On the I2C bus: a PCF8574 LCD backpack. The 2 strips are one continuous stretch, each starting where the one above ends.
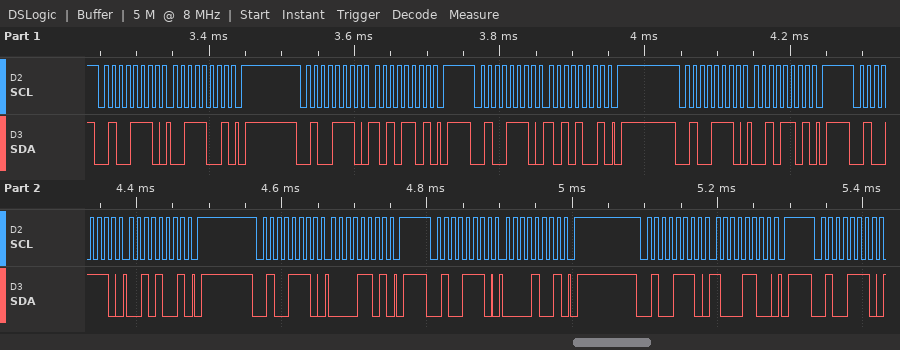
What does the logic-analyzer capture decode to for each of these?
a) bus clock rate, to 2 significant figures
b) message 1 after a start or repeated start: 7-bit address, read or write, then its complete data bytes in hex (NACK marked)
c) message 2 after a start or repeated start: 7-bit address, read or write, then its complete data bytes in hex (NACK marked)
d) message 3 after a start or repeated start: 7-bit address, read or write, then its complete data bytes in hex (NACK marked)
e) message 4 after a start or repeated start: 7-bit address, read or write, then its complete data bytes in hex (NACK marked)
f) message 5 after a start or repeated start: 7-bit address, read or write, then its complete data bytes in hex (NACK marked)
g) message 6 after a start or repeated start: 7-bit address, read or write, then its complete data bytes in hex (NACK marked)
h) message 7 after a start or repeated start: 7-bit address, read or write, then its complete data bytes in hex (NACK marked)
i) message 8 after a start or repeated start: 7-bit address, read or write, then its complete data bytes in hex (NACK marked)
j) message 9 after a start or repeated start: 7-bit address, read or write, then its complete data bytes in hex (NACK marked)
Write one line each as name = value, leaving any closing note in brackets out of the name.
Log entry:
bus clock rate, to 2 significant figures = 100 kHz
message 1 after a start or repeated start: 7-bit address, read or write, then its complete data bytes in hex = 0x27 write: 39
message 2 after a start or repeated start: 7-bit address, read or write, then its complete data bytes in hex = 0x27 write: AD
message 3 after a start or repeated start: 7-bit address, read or write, then its complete data bytes in hex = 0x27 write: A9
message 4 after a start or repeated start: 7-bit address, read or write, then its complete data bytes in hex = 0x27 write: 2D
message 5 after a start or repeated start: 7-bit address, read or write, then its complete data bytes in hex = 0x27 write: 29
message 6 after a start or repeated start: 7-bit address, read or write, then its complete data bytes in hex = 0x27 write: 0D
message 7 after a start or repeated start: 7-bit address, read or write, then its complete data bytes in hex = 0x27 write: 09
message 8 after a start or repeated start: 7-bit address, read or write, then its complete data bytes in hex = 0x27 write: 8C
message 9 after a start or repeated start: 7-bit address, read or write, then its complete data bytes in hex = 0x27 write
